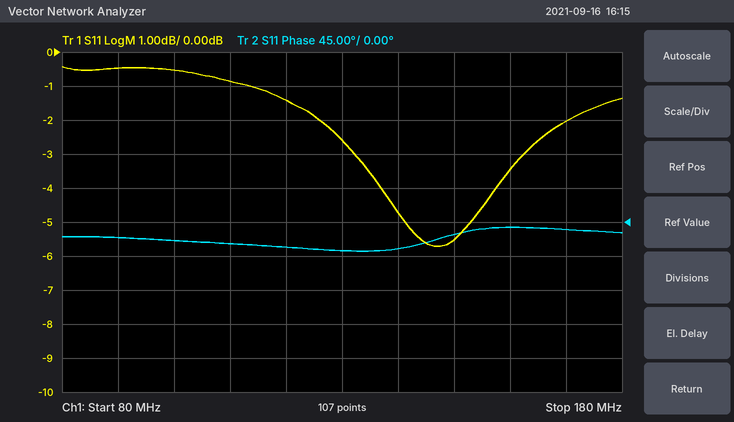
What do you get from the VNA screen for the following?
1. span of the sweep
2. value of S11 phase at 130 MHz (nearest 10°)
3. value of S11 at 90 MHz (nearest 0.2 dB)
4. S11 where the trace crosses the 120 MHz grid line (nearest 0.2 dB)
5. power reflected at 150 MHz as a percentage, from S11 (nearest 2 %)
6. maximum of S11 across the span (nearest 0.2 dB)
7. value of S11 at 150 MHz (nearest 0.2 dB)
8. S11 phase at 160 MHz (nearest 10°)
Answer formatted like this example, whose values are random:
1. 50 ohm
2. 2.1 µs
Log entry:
1. 100 MHz
2. -40°
3. -0.4 dB
4. -1.4 dB
5. 28 %
6. -0.4 dB
7. -5.6 dB
8. -10°
